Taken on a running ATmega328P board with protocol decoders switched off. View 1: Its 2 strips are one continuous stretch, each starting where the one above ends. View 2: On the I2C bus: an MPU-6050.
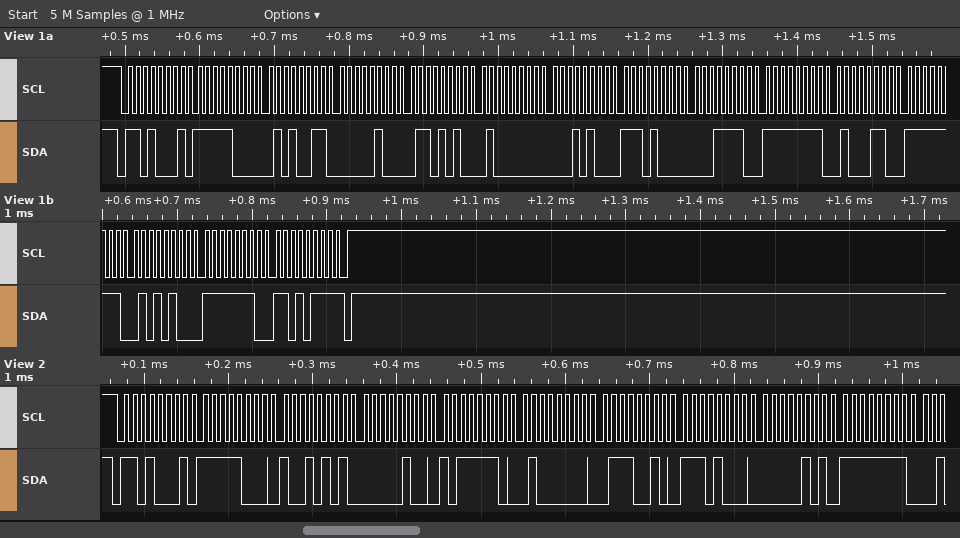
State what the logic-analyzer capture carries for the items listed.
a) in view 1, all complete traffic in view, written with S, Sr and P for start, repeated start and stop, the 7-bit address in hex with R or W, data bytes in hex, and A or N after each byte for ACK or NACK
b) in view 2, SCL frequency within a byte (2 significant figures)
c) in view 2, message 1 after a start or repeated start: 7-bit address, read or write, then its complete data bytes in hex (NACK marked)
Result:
S 68R A F8 A 53 A 04 A 6A A 40 A 14 A E8 A 1E A FF A 46 A FF A 54 A FE A D7 N P
100 kHz
0x68 read: F8 95 04 BE 40 72 E8 05 FF
